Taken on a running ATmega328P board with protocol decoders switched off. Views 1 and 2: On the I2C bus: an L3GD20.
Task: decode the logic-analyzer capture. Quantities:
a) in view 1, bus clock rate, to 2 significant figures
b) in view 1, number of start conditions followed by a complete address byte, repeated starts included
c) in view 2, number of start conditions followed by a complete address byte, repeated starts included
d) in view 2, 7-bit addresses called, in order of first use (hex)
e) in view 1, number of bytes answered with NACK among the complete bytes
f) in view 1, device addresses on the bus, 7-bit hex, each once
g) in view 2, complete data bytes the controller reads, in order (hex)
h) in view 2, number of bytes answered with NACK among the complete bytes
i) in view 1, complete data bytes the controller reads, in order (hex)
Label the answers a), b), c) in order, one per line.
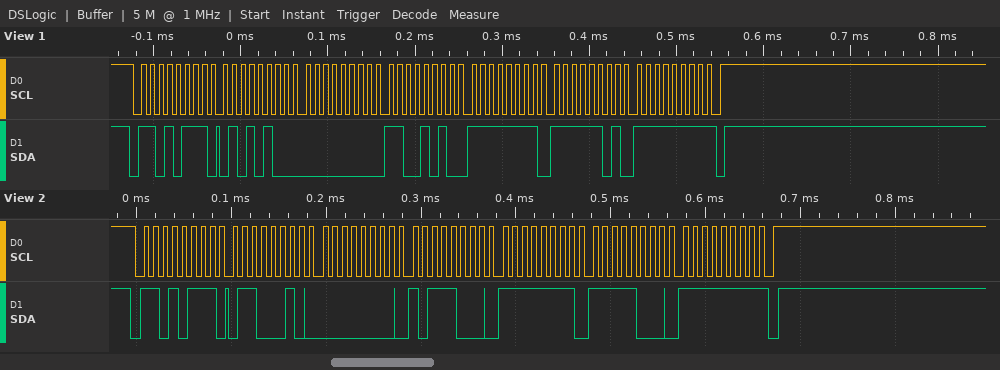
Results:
a) 100 kHz
b) 1
c) 1
d) 0x6B
e) 1
f) 0x6B
g) 62 00 B8 FF F8 FF
h) 1
i) 54 00 CA FF FD FF
